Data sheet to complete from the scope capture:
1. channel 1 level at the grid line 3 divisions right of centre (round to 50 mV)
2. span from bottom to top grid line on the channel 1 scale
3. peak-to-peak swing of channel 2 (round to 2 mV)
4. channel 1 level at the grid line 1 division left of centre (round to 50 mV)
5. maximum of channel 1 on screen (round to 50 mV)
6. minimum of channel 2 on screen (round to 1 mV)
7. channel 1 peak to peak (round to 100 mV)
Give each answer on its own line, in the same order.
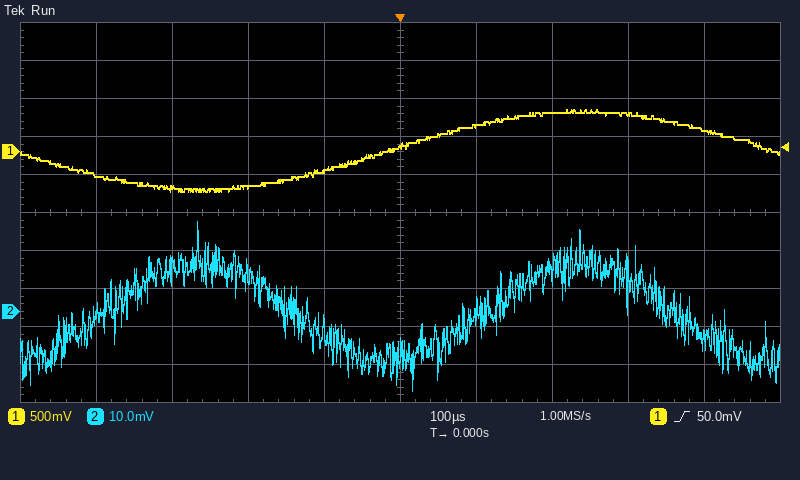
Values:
500 mV
5 V
44 mV
-250 mV
550 mV
-21 mV
1.10 V
